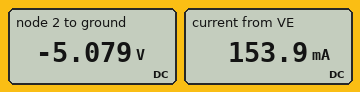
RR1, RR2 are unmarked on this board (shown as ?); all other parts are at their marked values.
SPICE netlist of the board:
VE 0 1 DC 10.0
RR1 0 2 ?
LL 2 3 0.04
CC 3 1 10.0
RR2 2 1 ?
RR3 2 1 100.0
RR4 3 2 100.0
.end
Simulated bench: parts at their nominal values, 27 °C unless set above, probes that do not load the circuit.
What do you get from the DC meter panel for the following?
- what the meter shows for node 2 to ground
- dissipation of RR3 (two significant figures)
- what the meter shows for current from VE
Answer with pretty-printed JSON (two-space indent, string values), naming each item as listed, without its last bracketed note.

{
  "what the meter shows for node 2 to ground": "-5.079 V",
  "dissipation of RR3": "240 mW",
  "what the meter shows for current from VE": "153.9 mA"
}
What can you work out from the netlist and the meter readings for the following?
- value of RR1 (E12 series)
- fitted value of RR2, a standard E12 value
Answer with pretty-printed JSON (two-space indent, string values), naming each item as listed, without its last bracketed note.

{
  "value of RR1": "33 Ω",
  "fitted value of RR2, a standard E12 value": "47 Ω"
}
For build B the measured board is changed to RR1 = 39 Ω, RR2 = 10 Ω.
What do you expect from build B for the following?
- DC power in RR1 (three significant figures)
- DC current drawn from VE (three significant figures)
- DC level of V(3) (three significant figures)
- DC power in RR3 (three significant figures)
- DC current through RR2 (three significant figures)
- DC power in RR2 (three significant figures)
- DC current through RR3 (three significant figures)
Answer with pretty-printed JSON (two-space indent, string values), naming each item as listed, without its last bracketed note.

{
  "DC power in RR1": "1.69 W",
  "DC current drawn from VE": "208 mA",
  "DC level of V(3)": "-8.11 V",
  "DC power in RR3": "35.7 mW",
  "DC current through RR2": "189 mA",
  "DC power in RR2": "357 mW",
  "DC current through RR3": "18.9 mA"
}
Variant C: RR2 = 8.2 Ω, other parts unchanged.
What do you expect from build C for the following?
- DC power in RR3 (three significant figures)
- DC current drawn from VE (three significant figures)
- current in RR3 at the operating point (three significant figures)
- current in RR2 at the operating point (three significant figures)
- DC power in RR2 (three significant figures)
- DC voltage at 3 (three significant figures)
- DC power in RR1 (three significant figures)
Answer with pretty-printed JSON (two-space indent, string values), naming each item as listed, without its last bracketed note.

{
  "DC power in RR3": "34.9 mW",
  "DC current drawn from VE": "246 mA",
  "current in RR3 at the operating point": "18.7 mA",
  "current in RR2 at the operating point": "228 mA",
  "DC power in RR2": "425 mW",
  "DC voltage at 3": "-8.13 V",
  "DC power in RR1": "2.00 W"
}
